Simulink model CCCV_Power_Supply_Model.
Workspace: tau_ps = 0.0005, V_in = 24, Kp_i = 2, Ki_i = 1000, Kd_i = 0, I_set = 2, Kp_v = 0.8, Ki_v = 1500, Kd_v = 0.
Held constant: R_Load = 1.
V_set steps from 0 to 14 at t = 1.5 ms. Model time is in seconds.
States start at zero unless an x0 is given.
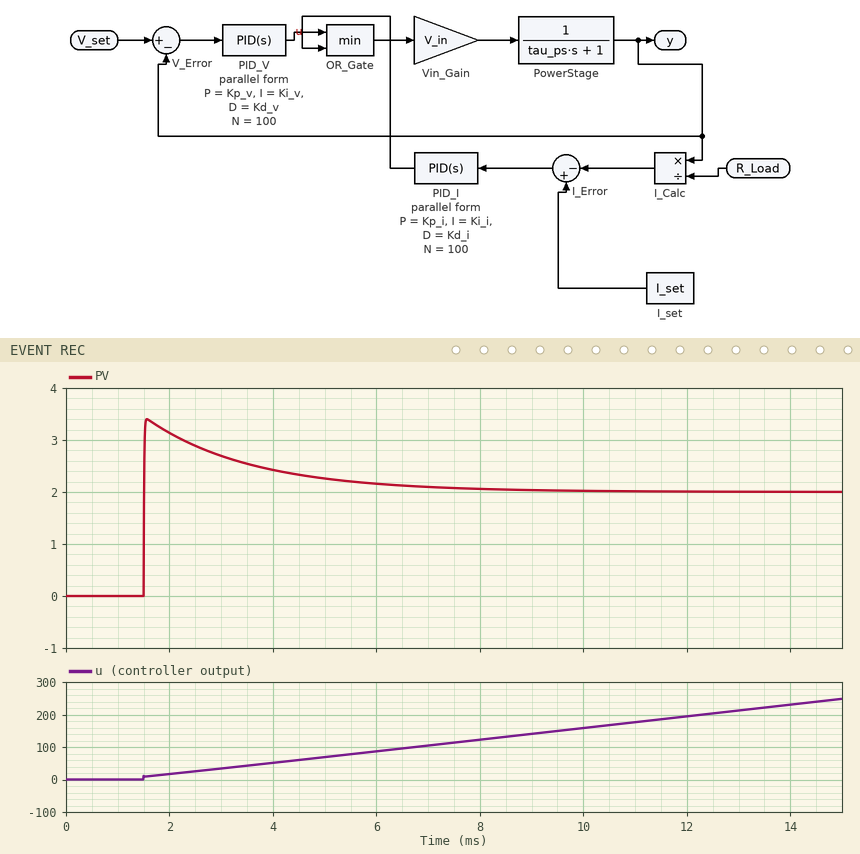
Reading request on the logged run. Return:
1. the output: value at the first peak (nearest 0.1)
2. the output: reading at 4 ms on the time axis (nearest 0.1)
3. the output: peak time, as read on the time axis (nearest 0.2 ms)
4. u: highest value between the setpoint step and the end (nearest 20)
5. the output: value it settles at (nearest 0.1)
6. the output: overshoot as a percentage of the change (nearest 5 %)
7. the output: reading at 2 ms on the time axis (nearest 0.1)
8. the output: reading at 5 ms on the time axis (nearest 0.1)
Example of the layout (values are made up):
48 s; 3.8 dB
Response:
3.4; 2.4; 1.6 ms; 240; 2.0; 70 %; 3.1; 2.3
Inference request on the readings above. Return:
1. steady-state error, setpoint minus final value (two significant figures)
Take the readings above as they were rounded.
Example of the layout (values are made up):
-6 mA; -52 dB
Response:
12
